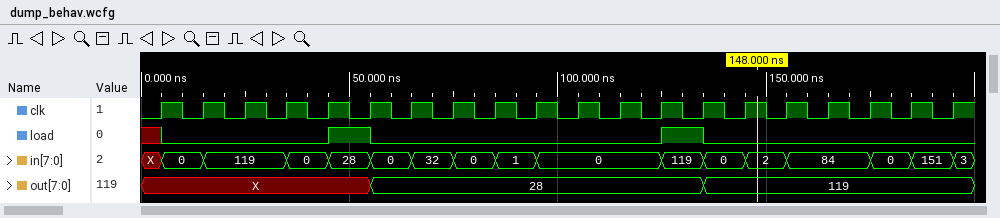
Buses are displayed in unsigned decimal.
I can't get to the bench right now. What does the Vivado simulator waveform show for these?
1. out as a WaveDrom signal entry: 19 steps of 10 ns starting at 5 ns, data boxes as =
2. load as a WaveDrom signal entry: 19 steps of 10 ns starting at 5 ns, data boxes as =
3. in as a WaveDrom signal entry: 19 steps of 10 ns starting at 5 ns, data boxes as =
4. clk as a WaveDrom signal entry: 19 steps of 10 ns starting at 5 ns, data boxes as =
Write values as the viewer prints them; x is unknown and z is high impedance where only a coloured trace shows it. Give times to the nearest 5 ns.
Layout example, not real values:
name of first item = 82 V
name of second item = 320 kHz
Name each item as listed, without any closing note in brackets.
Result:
out as a WaveDrom signal entry: 19 steps of 10 ns starting at 5 ns, data boxes as = = {name: 'out', wave: 'x....=.......=.....', data: '28 119'}
load as a WaveDrom signal entry: 19 steps of 10 ns starting at 5 ns, data boxes as = = {name: 'load', wave: '0...10......10.....'}
in as a WaveDrom signal entry: 19 steps of 10 ns starting at 5 ns, data boxes as = = {name: 'in', wave: '==.=======..====.==', data: '0 119 0 28 0 32 0 1 0 119 0 2 84 0 151'}
clk as a WaveDrom signal entry: 19 steps of 10 ns starting at 5 ns, data boxes as = = {name: 'clk', wave: 'p..................'}
